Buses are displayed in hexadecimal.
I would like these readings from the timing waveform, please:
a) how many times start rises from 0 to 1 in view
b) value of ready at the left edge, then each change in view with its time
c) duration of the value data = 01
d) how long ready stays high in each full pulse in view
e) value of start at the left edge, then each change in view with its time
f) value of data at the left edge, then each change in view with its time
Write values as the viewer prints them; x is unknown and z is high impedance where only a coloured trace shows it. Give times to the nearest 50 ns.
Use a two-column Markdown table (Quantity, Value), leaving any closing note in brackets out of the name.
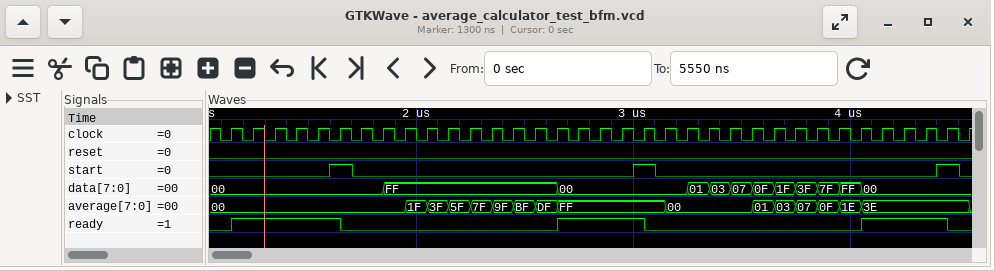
| Quantity | Value |
|---|---|
| how many times start rises from 0 to 1 in view | 3 |
| value of ready at the left edge, then each change in view with its time | 0, 1 at 1150 ns, 0 at 1650 ns, 1 at 2650 ns, 0 at 3050 ns, 1 at 4050 ns, 0 at 4450 ns |
| duration of the value data = 01 | 100 ns |
| how long ready stays high in each full pulse in view | 500 ns, 400 ns, 400 ns |
| value of start at the left edge, then each change in view with its time | 0, 1 at 1600 ns, 0 at 1700 ns, 1 at 3000 ns, 0 at 3100 ns, 1 at 4400 ns, 0 at 4500 ns |
| value of data at the left edge, then each change in view with its time | 00, FF at 1850 ns, 00 at 2650 ns, 01 at 3250 ns, 03 at 3350 ns, 07 at 3450 ns, 0F at 3550 ns, 1F at 3650 ns, 3F at 3750 ns, 7F at 3850 ns, FF at 3950 ns, 00 at 4050 ns |
